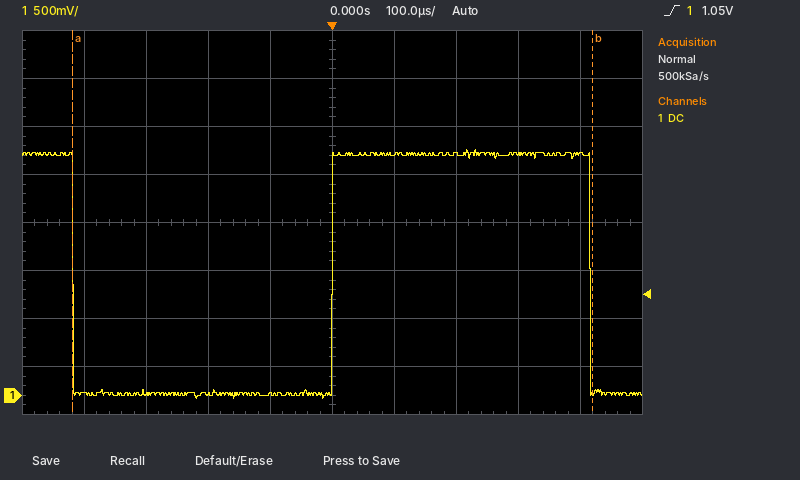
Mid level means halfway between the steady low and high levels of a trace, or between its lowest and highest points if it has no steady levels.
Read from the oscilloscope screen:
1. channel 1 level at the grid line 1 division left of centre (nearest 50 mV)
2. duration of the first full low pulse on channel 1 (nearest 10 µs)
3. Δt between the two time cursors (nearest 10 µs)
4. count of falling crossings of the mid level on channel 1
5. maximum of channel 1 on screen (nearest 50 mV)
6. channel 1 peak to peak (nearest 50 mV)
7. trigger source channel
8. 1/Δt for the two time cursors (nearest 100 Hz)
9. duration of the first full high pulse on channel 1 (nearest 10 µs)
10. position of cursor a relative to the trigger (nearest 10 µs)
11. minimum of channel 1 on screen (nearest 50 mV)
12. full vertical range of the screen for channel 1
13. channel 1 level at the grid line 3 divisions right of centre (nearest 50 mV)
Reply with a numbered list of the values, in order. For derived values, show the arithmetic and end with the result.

1. 0 mV
2. 420 µs
3. 840 µs
4. 2
5. 2.55 V
6. 2.55 V − (-50 mV) = 2.60 V
7. channel 1
8. 1 / 840 µs ≈ 1.2 kHz
9. 420 µs
10. -420 µs
11. -50 mV
12. 4 V
13. 2.50 V
